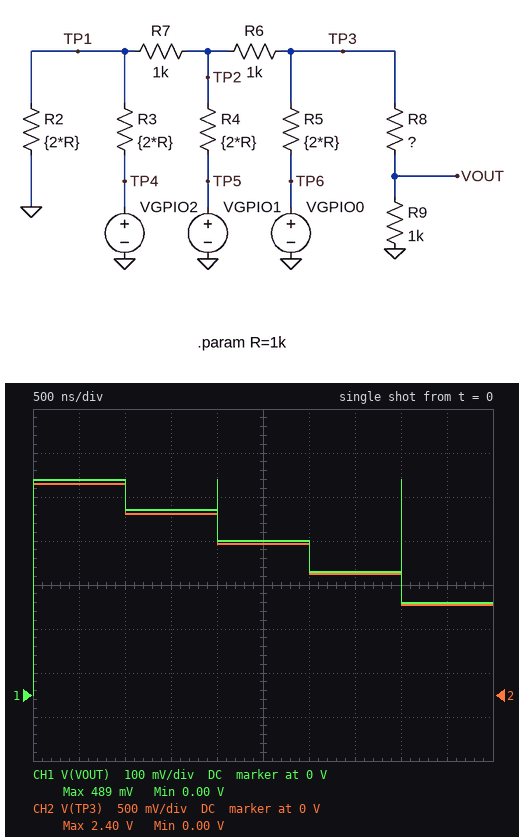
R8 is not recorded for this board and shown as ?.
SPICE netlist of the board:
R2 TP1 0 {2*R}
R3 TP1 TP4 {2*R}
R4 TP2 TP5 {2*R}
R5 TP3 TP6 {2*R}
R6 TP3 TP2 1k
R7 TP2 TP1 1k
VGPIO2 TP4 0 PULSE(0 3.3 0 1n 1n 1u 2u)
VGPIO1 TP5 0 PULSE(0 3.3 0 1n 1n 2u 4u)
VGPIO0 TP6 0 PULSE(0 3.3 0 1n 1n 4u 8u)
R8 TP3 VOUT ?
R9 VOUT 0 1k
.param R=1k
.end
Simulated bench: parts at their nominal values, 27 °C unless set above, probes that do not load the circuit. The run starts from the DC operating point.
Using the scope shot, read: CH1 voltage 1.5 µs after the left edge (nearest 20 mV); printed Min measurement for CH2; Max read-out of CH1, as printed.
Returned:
420 mV
0.00 V
489 mV
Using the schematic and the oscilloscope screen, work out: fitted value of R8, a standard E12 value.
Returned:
3.9 kΩ
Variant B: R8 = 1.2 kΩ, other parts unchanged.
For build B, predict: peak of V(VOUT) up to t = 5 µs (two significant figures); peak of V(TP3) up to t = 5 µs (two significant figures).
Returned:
900 mV
2.0 V
